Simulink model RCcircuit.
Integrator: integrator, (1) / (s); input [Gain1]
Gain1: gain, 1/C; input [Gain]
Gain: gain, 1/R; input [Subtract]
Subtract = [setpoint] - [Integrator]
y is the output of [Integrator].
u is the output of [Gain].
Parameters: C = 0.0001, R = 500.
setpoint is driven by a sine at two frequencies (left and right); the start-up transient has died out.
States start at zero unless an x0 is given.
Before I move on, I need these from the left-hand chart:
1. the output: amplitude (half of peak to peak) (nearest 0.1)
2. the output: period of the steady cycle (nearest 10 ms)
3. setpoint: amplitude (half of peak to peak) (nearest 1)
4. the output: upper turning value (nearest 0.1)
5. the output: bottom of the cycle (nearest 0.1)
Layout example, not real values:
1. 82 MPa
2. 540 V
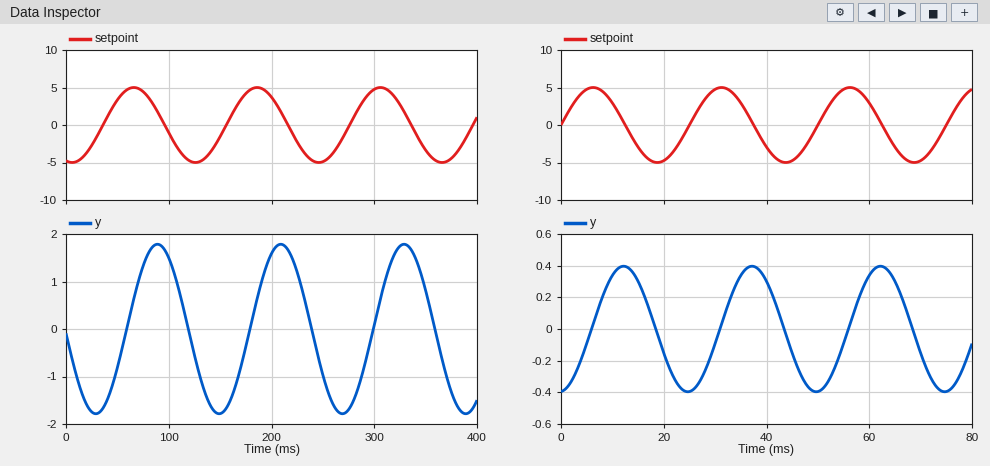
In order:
1. 1.8
2. 120 ms
3. 5
4. 1.8
5. -1.8
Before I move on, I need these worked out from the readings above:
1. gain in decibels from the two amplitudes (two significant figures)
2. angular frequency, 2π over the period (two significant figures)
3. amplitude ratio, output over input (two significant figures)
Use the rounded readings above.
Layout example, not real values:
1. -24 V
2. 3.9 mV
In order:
1. -8.9 dB
2. 0.052 rad/ms
3. 0.36
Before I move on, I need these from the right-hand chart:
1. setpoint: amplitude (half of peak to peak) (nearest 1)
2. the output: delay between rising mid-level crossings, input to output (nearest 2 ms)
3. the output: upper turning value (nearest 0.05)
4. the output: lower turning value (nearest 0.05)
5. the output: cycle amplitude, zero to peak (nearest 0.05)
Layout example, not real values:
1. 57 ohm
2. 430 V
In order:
1. 5
2. 6 ms
3. 0.40
4. -0.40
5. 0.40
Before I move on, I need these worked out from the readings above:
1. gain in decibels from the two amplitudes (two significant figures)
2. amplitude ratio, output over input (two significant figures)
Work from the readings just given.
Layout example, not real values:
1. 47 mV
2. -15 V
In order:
1. -22 dB
2. 0.080
